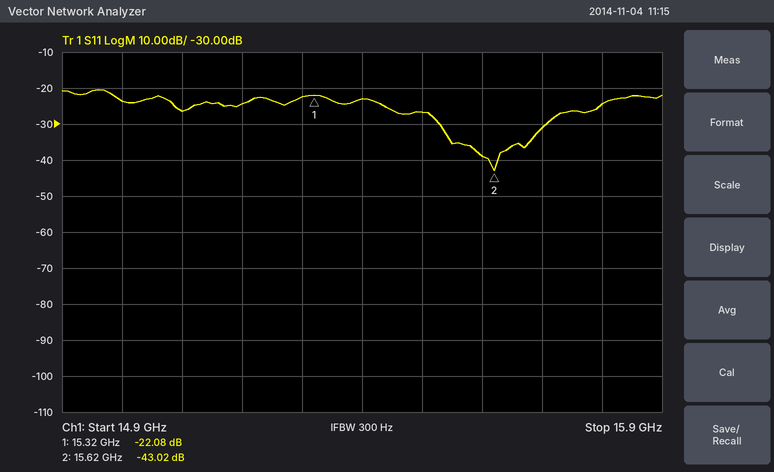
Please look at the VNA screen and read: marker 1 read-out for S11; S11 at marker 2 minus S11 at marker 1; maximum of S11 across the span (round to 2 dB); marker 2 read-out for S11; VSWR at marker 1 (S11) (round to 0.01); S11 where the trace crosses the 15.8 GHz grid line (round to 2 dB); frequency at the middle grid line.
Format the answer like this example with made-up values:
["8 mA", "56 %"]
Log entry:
["-22.08 dB", "-20.94 dB", "-20 dB", "-43.02 dB", "1.17", "-24 dB", "15.4 GHz"]
